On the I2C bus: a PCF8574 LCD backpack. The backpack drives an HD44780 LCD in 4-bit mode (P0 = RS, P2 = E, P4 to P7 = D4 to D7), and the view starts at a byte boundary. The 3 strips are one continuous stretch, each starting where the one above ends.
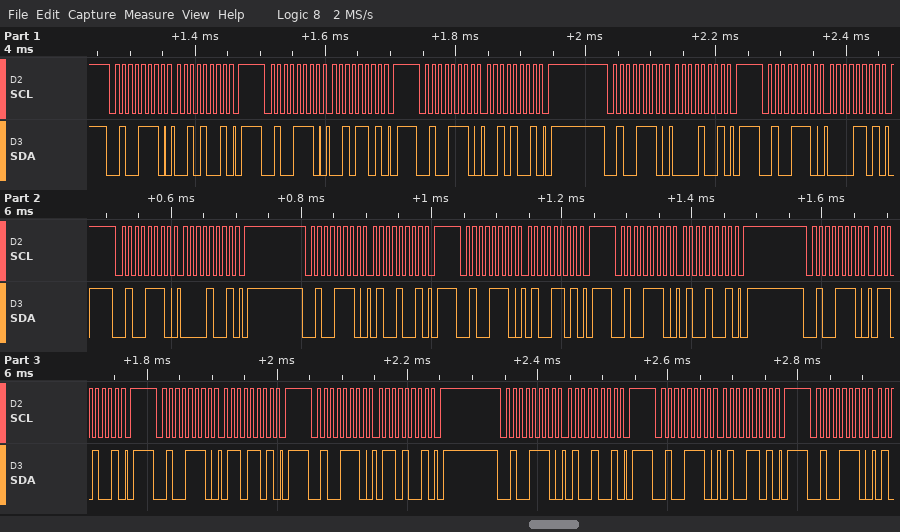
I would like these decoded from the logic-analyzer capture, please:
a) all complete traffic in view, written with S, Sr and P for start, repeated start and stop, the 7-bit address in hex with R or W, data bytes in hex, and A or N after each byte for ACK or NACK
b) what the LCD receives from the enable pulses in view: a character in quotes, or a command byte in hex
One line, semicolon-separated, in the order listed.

S 27W A 29 A P S 27W A 2D A P S 27W A 29 A P S 27W A 09 A P S 27W A 0D A P S 27W A 09 A P S 27W A 49 A P S 27W A 4D A P S 27W A 49 A P S 27W A 69 A P S 27W A 6D A P S 27W A 69 A P S 27W A 49 A P S 27W A 4D A P S 27W A; ' ' 'F'
